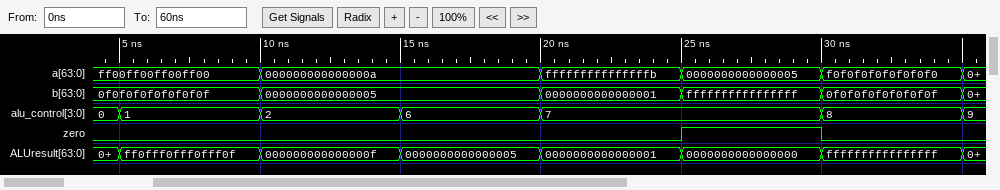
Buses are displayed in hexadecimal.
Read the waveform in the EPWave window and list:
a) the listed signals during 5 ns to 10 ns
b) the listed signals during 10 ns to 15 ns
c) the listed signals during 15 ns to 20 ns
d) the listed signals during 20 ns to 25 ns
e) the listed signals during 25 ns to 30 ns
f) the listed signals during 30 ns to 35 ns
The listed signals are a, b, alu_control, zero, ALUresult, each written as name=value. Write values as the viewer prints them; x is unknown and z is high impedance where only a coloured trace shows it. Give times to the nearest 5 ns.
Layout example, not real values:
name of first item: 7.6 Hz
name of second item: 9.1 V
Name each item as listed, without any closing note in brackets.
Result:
the listed signals during 5 ns to 10 ns: a=ff00ff00ff00ff00, b=0f0f0f0f0f0f0f0f, alu_control=1, zero=0, ALUresult=ff0fff0fff0fff0f
the listed signals during 10 ns to 15 ns: a=000000000000000a, b=0000000000000005, alu_control=2, zero=0, ALUresult=000000000000000f
the listed signals during 15 ns to 20 ns: a=000000000000000a, b=0000000000000005, alu_control=6, zero=0, ALUresult=0000000000000005
the listed signals during 20 ns to 25 ns: a=fffffffffffffffb, b=0000000000000001, alu_control=7, zero=0, ALUresult=0000000000000001
the listed signals during 25 ns to 30 ns: a=0000000000000005, b=ffffffffffffffff, alu_control=7, zero=1, ALUresult=0000000000000000
the listed signals during 30 ns to 35 ns: a=f0f0f0f0f0f0f0f0, b=0f0f0f0f0f0f0f0f, alu_control=8, zero=0, ALUresult=ffffffffffffffff
